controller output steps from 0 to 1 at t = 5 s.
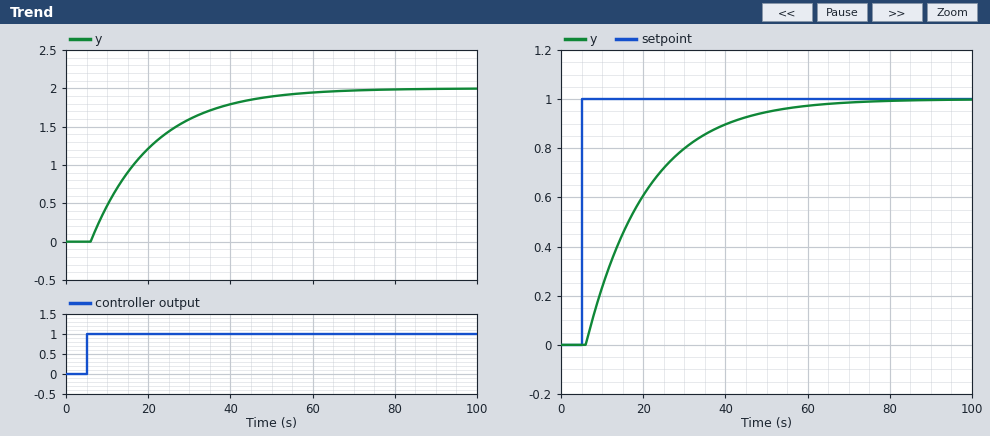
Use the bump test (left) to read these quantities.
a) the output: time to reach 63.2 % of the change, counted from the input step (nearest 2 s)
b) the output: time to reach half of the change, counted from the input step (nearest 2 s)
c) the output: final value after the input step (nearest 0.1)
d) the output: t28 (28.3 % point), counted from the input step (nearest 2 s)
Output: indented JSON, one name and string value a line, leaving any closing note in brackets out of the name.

{
  "the output: time to reach 63.2 % of the change, counted from the input step": "16 s",
  "the output: time to reach half of the change, counted from the input step": "12 s",
  "the output: final value after the input step": "2.0",
  "the output: t28 (28.3 % point), counted from the input step": "6 s"
}
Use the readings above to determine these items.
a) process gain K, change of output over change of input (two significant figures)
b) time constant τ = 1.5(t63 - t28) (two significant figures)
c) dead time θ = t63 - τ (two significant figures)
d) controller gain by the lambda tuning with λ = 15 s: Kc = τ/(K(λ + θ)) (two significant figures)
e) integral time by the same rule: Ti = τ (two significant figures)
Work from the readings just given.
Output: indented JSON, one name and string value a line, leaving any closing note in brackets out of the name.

{
  "process gain K, change of output over change of input": "2.0",
  "time constant τ = 1.5(t63 - t28)": "15 s",
  "dead time θ = t63 - τ": "1.0 s",
  "controller gain by the lambda tuning with λ = 15 s: Kc = τ/(K(λ + θ))": "0.47",
  "integral time by the same rule: Ti = τ": "15 s"
}
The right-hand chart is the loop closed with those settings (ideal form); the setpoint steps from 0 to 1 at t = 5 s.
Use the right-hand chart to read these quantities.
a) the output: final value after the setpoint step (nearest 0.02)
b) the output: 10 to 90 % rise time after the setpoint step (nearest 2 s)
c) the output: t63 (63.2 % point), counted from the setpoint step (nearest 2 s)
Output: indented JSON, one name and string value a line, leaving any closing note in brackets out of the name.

{
  "the output: final value after the setpoint step": "1.00",
  "the output: 10 to 90 % rise time after the setpoint step": "32 s",
  "the output: t63 (63.2 % point), counted from the setpoint step": "16 s"
}
